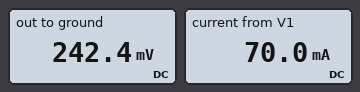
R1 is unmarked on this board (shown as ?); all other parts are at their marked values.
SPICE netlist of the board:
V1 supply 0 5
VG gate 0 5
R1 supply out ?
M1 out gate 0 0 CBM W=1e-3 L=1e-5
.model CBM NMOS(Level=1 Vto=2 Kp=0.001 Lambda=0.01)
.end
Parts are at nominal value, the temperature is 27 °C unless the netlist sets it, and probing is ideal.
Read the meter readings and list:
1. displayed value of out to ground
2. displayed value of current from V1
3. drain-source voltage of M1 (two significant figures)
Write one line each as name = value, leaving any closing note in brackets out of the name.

displayed value of out to ground = 242.4 mV
displayed value of current from V1 = 70.0 mA
drain-source voltage of M1 = 240 mV
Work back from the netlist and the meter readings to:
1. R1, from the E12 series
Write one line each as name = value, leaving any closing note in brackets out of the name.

R1, from the E12 series = 68 Ω
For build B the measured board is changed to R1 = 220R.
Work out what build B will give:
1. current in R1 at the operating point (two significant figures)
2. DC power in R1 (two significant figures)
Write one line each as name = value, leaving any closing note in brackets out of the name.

current in R1 at the operating point = 22 mA
DC power in R1 = 110 mW
